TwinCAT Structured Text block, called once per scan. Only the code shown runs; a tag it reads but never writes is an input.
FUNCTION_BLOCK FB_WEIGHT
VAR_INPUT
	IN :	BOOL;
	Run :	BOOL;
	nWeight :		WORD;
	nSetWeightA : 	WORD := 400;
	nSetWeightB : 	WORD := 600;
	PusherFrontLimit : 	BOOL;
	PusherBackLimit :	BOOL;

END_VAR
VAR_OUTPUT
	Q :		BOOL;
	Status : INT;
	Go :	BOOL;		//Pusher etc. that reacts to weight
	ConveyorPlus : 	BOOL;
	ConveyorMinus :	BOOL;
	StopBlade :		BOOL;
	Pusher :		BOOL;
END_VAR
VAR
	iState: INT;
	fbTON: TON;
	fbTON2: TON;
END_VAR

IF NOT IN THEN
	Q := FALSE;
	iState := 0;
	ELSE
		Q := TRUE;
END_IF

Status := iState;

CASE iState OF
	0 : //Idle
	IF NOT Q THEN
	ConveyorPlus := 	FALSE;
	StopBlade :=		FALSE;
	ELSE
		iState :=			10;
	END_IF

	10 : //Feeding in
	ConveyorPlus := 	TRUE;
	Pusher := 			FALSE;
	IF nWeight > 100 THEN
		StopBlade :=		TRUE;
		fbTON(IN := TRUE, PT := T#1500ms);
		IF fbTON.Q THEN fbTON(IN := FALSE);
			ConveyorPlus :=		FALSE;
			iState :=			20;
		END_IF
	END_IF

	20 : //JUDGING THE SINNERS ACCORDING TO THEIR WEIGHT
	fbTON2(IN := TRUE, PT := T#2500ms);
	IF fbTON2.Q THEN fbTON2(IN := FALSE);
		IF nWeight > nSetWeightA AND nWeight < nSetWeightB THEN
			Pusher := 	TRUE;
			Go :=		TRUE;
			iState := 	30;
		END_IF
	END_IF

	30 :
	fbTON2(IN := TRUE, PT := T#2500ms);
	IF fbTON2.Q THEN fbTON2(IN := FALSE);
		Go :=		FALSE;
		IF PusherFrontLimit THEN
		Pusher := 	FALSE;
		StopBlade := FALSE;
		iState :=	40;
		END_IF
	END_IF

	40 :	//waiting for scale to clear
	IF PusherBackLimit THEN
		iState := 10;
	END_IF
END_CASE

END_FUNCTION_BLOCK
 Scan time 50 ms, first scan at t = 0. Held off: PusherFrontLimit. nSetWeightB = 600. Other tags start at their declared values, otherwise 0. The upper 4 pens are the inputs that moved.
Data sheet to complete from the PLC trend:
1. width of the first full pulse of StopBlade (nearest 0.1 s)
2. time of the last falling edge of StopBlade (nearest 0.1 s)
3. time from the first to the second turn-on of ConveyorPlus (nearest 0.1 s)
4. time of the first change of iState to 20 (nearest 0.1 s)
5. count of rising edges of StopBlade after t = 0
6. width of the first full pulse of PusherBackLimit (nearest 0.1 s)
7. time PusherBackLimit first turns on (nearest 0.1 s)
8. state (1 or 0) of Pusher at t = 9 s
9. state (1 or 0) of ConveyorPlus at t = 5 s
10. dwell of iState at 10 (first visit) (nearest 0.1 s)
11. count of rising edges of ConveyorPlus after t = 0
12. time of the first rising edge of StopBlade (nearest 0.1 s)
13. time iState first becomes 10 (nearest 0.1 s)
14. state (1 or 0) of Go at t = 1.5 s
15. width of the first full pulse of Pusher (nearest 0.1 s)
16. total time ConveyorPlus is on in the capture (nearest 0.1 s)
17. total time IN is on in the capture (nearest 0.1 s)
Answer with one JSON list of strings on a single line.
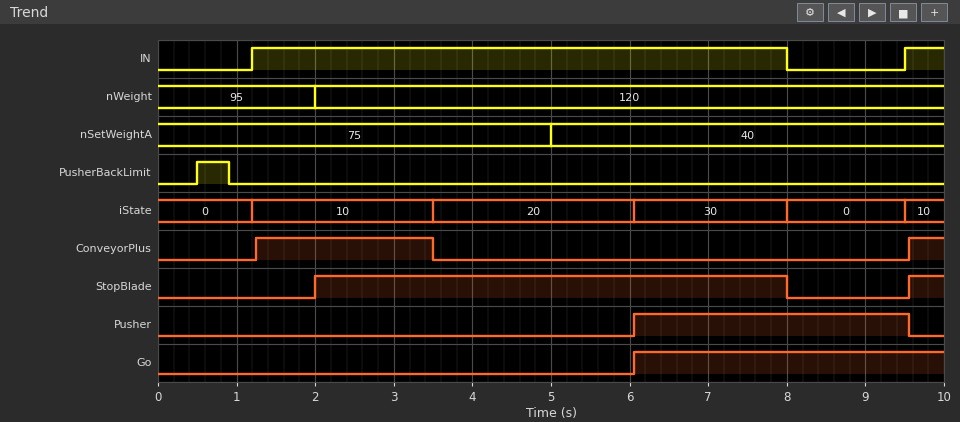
["6.0 s", "8.0 s", "8.3 s", "3.5 s", "2", "0.4 s", "0.5 s", "1", "0", "2.3 s", "2", "2.0 s", "1.2 s", "0", "3.5 s", "2.7 s", "7.3 s"]
